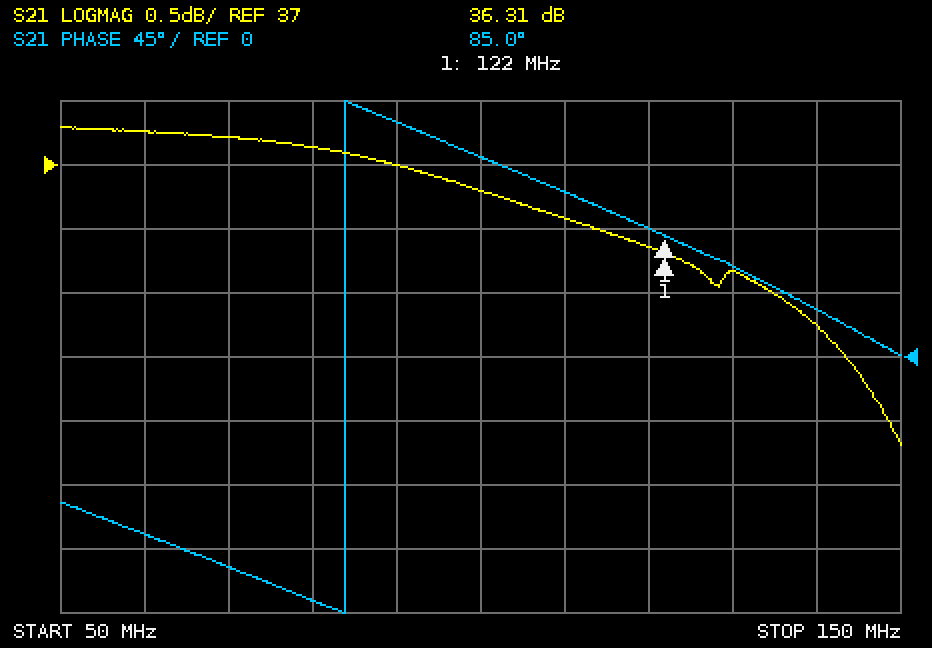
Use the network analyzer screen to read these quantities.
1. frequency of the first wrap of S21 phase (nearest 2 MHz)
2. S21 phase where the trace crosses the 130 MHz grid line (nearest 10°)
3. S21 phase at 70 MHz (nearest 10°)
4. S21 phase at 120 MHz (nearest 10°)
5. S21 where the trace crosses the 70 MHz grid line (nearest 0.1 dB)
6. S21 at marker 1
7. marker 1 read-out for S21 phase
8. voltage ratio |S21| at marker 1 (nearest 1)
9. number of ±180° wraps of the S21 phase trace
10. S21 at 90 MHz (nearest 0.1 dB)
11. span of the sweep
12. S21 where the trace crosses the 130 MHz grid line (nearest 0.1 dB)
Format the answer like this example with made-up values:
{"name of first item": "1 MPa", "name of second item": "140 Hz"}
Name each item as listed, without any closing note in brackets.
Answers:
{"frequency of the first wrap of S21 phase": "84 MHz", "S21 phase where the trace crosses the 130 MHz grid line": "60°", "S21 phase at 70 MHz": "-150°", "S21 phase at 120 MHz": "90°", "S21 where the trace crosses the 70 MHz grid line": "37.2 dB", "S21 at marker 1": "36.31 dB", "marker 1 read-out for S21 phase": "85.0°", "voltage ratio |S21| at marker 1": "65", "number of ±180° wraps of the S21 phase trace": "1", "S21 at 90 MHz": "37.0 dB", "span of the sweep": "100 MHz", "S21 where the trace crosses the 130 MHz grid line": "36.2 dB"}
